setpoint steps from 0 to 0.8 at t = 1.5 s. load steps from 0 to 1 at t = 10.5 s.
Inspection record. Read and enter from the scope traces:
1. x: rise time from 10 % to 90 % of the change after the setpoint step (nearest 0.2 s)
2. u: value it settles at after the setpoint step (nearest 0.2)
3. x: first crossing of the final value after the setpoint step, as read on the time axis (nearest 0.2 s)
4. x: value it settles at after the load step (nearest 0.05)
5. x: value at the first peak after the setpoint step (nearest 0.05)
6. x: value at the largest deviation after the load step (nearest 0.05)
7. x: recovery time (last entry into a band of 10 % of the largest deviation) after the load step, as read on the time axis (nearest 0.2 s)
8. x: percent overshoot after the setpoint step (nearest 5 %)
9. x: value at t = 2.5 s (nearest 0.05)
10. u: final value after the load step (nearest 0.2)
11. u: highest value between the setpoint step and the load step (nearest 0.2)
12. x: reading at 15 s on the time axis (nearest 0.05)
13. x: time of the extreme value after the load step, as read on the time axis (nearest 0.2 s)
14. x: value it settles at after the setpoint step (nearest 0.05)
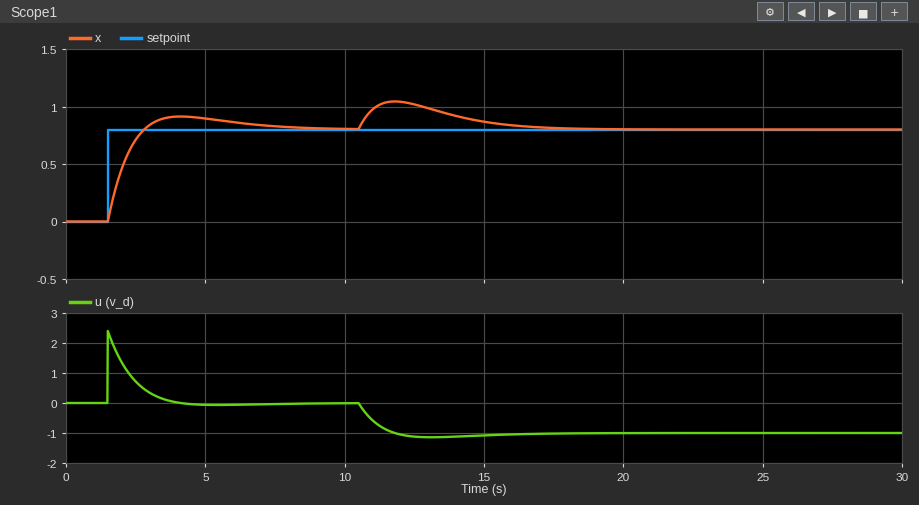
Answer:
1.0 s
0.0
2.8 s
0.80
0.90
1.05
16.6 s
15 %
0.70
-1.0
2.4
0.85
11.8 s
0.80
